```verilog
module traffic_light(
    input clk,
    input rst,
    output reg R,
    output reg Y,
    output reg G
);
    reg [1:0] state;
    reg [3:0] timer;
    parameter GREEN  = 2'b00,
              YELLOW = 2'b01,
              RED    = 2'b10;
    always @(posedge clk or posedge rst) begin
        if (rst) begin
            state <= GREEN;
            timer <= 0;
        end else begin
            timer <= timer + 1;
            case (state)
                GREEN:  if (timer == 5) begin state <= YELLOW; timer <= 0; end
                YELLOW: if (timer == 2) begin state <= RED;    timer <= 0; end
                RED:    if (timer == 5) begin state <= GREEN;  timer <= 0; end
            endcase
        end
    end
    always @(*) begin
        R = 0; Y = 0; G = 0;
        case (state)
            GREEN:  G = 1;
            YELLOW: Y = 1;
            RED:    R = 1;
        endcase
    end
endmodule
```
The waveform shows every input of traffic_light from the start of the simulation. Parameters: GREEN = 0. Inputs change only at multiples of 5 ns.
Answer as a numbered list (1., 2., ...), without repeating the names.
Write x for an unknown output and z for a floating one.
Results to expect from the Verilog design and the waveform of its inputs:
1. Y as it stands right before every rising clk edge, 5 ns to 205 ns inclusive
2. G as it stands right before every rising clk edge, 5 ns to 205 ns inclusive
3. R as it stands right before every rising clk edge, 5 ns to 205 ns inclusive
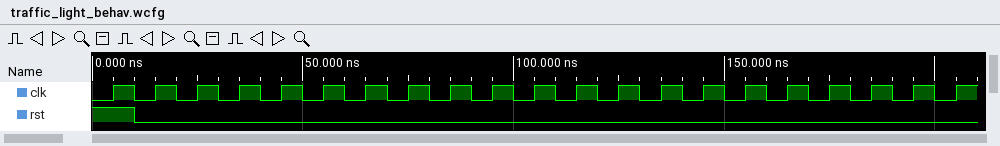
1. 0 0 0 0 0 0 0 1 1 1 0 0 0 0 0 0 0 0 0 0 0
2. 1 1 1 1 1 1 1 0 0 0 0 0 0 0 0 0 1 1 1 1 1
3. 0 0 0 0 0 0 0 0 0 0 1 1 1 1 1 1 0 0 0 0 0
